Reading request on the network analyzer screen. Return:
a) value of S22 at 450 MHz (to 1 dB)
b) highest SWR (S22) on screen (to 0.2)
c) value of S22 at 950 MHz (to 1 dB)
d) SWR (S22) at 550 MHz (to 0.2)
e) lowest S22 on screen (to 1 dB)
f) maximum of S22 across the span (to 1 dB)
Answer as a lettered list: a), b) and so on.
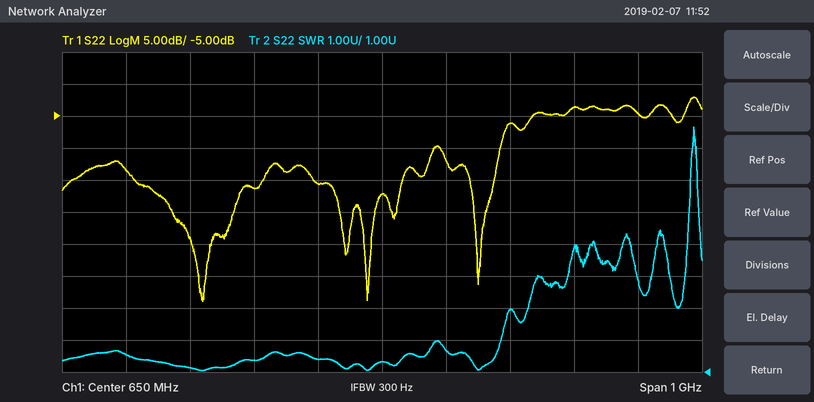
a) -16 dB
b) 8.6
c) -4 dB
d) 1.4
e) -34 dB
f) -2 dB
